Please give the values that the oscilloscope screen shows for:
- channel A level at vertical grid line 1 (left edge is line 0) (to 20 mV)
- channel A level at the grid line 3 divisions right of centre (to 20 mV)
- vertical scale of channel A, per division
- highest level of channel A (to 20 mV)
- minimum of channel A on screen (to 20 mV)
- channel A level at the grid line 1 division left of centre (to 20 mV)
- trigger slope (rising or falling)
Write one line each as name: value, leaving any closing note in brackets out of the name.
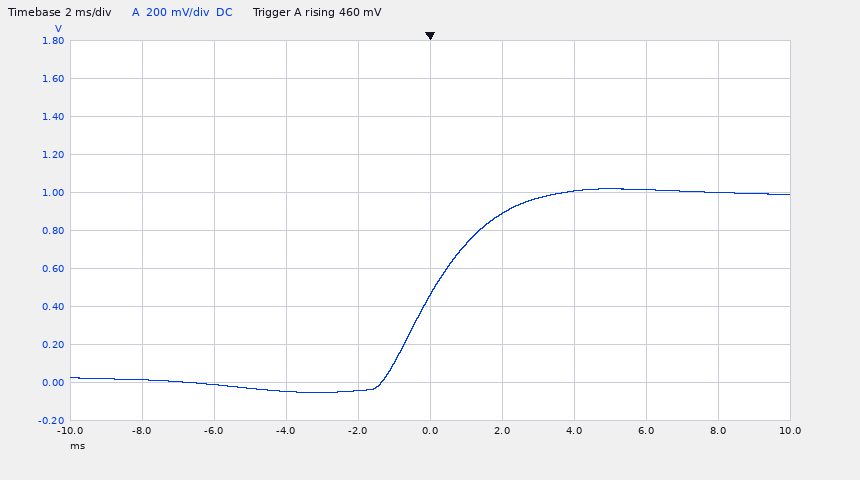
channel A level at vertical grid line 1 (left edge is line 0): 20 mV
channel A level at the grid line 3 divisions right of centre: 1.02 V
vertical scale of channel A, per division: 200 mV
highest level of channel A: 1.02 V
minimum of channel A on screen: -60 mV
channel A level at the grid line 1 division left of centre: -40 mV
trigger slope: rising
